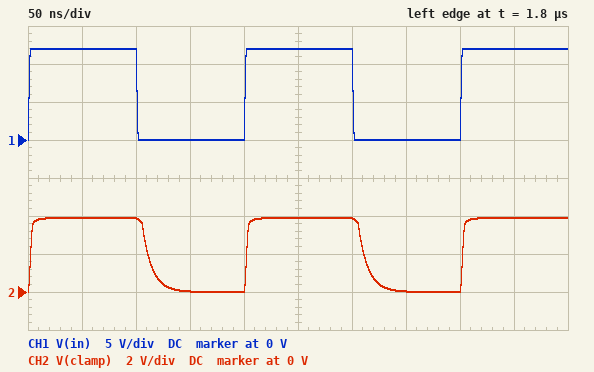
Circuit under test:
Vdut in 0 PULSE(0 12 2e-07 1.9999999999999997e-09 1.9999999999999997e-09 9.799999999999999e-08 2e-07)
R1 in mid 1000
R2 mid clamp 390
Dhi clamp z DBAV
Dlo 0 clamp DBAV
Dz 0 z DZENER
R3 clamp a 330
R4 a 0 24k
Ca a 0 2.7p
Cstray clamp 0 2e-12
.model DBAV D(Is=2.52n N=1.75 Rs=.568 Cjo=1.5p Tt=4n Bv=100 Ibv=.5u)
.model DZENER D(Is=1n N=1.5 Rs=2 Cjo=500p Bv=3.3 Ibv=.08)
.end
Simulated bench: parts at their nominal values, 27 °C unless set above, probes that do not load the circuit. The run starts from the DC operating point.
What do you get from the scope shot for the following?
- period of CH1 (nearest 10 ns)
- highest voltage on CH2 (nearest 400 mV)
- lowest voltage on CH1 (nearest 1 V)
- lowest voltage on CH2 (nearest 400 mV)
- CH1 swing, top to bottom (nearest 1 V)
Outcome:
200 ns
4.0 V
0 V
0 V
12 V
